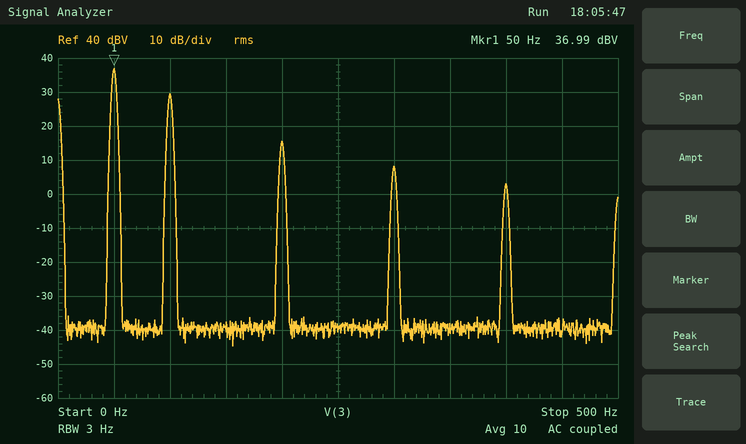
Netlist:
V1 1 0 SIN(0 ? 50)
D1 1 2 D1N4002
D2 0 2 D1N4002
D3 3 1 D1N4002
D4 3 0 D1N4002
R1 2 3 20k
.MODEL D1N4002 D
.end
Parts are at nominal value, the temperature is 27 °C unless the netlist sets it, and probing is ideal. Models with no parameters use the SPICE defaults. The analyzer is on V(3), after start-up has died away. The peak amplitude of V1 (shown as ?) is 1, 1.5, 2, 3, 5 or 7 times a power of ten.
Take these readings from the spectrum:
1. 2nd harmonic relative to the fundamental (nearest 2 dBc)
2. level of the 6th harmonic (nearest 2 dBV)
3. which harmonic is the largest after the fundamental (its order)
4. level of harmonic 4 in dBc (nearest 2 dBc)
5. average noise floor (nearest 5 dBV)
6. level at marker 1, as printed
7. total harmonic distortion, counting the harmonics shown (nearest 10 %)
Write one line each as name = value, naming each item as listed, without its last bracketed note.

2nd harmonic relative to the fundamental = -8 dBc
level of the 6th harmonic = 8 dBV
which harmonic is the largest after the fundamental = 2
level of harmonic 4 in dBc = -22 dBc
average noise floor = -40 dBV
level at marker 1, as printed = 36.99 dBV
total harmonic distortion, counting the harmonics shown = 40 %
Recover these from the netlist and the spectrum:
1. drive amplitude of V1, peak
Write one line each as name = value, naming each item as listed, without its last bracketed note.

drive amplitude of V1, peak = 200 V
